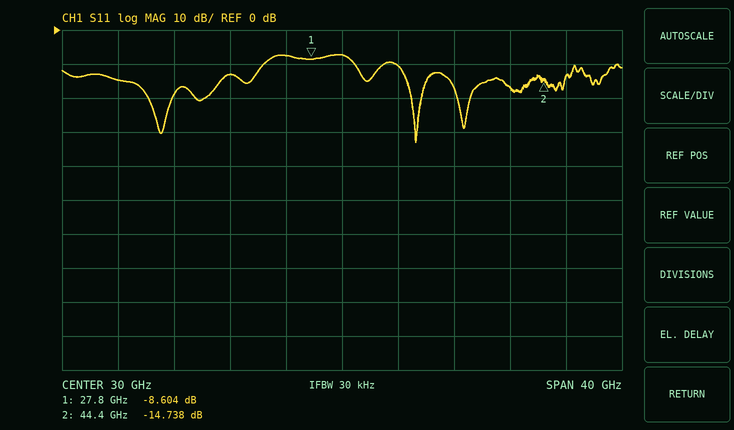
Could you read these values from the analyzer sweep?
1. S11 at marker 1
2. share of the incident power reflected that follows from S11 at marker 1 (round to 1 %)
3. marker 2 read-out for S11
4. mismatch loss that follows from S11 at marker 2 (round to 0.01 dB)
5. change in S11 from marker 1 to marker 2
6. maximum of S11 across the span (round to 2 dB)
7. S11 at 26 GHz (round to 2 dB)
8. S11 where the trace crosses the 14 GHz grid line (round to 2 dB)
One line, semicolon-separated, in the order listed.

-8.604 dB; 14 %; -14.738 dB; 0.15 dB; -6.134 dB; -8 dB; -8 dB; -14 dB
